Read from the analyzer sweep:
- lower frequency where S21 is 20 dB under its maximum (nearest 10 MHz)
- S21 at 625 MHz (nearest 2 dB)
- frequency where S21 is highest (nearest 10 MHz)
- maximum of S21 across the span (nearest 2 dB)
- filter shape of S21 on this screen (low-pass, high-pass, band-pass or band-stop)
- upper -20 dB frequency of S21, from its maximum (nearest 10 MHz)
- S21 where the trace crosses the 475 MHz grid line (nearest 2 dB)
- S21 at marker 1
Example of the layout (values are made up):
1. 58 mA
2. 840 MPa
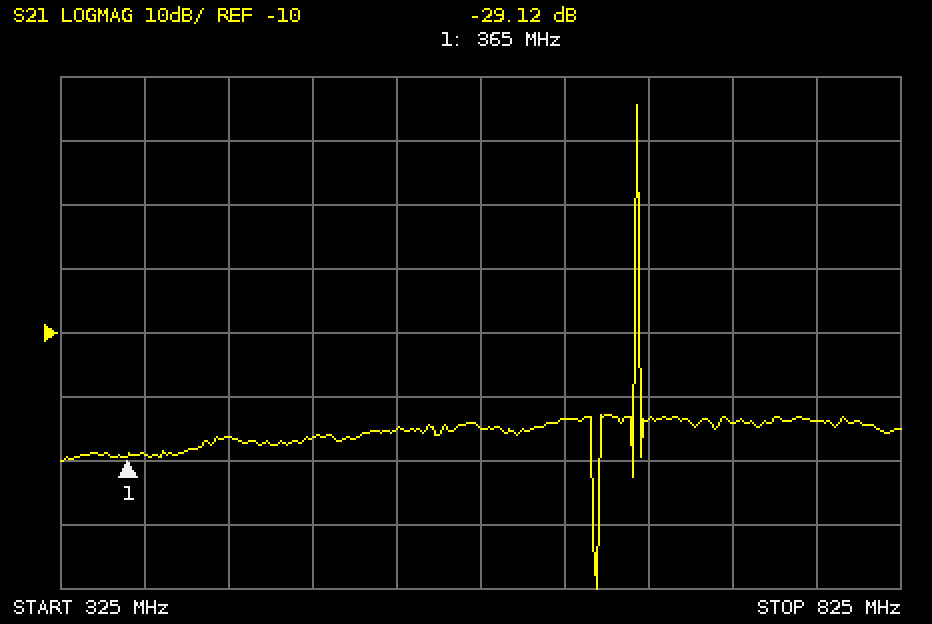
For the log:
1. 670 MHz
2. -24 dB
3. 670 MHz
4. 26 dB
5. band-pass
6. 670 MHz
7. -26 dB
8. -29.12 dB
